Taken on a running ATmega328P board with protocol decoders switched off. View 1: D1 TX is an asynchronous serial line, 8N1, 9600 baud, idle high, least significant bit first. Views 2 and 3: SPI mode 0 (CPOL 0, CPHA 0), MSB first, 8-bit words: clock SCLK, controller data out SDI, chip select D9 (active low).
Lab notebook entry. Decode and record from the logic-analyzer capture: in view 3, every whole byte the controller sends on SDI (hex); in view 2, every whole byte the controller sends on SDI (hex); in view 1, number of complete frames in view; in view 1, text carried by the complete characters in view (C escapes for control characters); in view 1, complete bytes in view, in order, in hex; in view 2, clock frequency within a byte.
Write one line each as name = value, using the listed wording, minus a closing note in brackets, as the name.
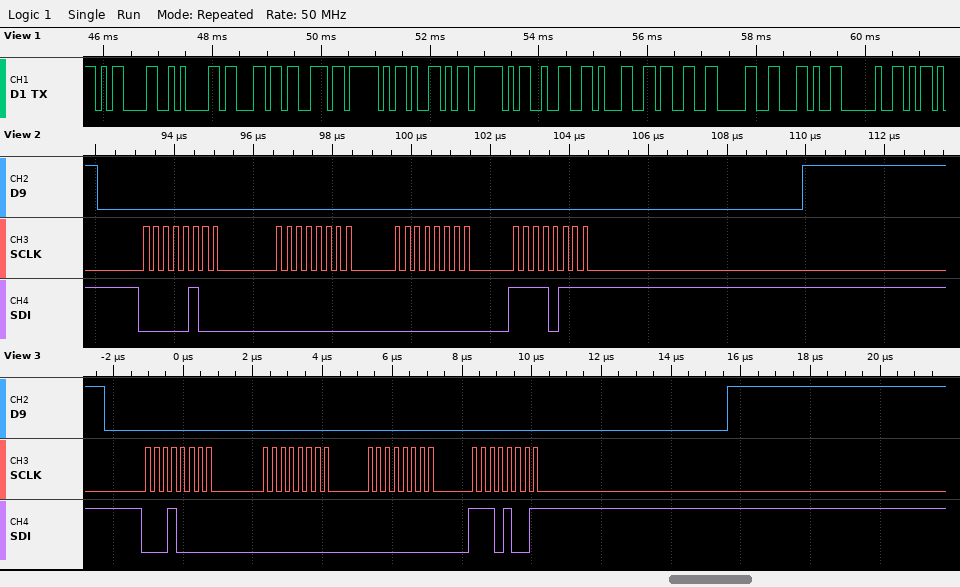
in view 3, every whole byte the controller sends on SDI = 10 00 00 E9
in view 2, every whole byte the controller sends on SDI = 0x04 0x00 0x00 0xF7
in view 1, number of complete frames in view = 13
in view 1, text carried by the complete characters in view = "\r\ncs_Y_2130, "
in view 1, complete bytes in view, in order, in hex = 0D 0A 63 73 5F 59 5F 32 31 33 30 2C 20
in view 2, clock frequency within a byte = 4 MHz
